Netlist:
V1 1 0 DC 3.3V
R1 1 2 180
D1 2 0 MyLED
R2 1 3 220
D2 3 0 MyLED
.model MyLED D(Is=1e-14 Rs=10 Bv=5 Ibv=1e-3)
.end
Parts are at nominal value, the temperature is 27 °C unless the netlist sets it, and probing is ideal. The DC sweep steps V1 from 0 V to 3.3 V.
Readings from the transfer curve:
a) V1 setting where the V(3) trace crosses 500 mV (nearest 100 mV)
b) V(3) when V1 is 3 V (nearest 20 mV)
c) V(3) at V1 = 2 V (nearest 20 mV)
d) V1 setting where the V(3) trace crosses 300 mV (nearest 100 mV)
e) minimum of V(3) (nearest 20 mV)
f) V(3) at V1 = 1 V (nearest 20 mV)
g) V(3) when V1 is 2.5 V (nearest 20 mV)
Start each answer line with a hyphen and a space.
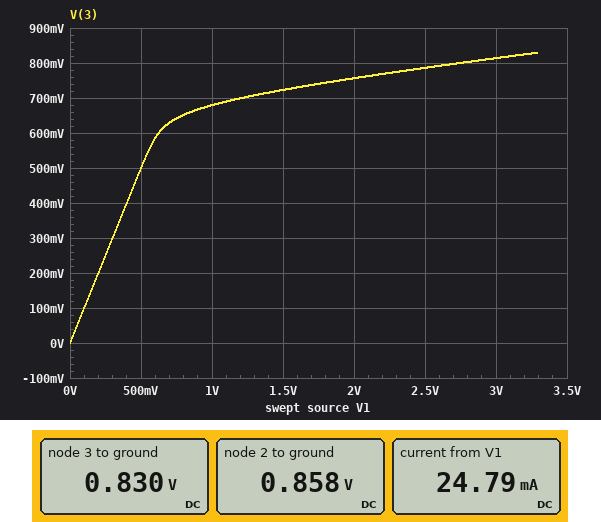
- 500 mV
- 820 mV
- 760 mV
- 300 mV
- 0 V
- 680 mV
- 780 mV
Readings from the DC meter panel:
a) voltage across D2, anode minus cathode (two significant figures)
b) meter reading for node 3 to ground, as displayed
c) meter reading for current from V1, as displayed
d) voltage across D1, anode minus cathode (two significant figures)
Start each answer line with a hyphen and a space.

- 830 mV
- 0.830 V
- 24.79 mA
- 860 mV
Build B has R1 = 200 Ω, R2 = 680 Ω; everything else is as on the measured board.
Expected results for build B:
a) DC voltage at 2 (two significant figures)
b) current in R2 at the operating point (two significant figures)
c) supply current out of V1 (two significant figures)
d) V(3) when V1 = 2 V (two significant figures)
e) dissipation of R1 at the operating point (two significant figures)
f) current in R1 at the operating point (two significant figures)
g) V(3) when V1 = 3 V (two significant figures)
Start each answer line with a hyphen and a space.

- 840 mV
- 3.8 mA
- 16 mA
- 690 mV
- 30 mW
- 12 mA
- 720 mV
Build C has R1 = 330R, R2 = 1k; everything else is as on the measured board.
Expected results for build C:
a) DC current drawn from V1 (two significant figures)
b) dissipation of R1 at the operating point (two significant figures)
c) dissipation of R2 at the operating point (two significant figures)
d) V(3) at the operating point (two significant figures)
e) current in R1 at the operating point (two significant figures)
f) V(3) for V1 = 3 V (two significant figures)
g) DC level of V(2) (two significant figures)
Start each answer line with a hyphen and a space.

- 10 mA
- 19 mW
- 6.7 mW
- 710 mV
- 7.6 mA
- 700 mV
- 780 mV
